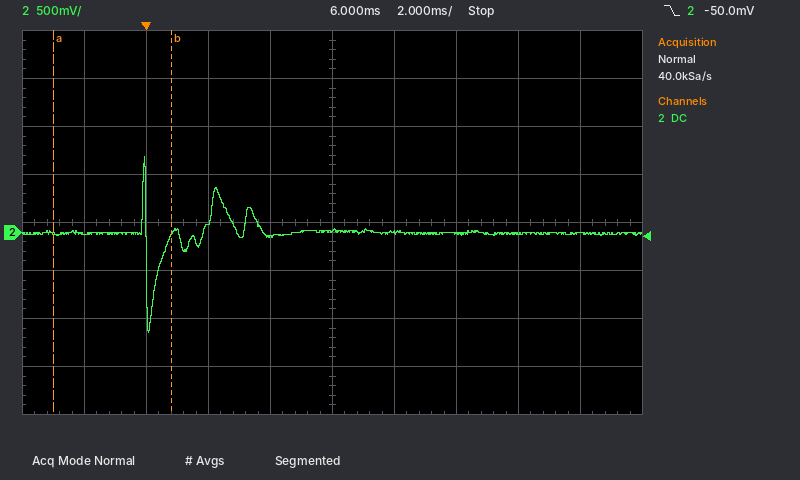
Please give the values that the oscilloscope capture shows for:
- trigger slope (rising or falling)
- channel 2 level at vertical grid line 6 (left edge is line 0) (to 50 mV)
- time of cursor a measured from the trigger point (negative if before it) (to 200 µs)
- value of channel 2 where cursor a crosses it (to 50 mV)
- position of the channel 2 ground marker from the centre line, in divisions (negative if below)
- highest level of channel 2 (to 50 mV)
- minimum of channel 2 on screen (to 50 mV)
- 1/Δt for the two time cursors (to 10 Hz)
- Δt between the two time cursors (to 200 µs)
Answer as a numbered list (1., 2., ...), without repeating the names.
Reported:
1. falling
2. 0 mV
3. -3.0 ms
4. 0 mV
5. -0.2 div
6. 800 mV
7. -1.05 V
8. 260 Hz
9. 3.8 ms
